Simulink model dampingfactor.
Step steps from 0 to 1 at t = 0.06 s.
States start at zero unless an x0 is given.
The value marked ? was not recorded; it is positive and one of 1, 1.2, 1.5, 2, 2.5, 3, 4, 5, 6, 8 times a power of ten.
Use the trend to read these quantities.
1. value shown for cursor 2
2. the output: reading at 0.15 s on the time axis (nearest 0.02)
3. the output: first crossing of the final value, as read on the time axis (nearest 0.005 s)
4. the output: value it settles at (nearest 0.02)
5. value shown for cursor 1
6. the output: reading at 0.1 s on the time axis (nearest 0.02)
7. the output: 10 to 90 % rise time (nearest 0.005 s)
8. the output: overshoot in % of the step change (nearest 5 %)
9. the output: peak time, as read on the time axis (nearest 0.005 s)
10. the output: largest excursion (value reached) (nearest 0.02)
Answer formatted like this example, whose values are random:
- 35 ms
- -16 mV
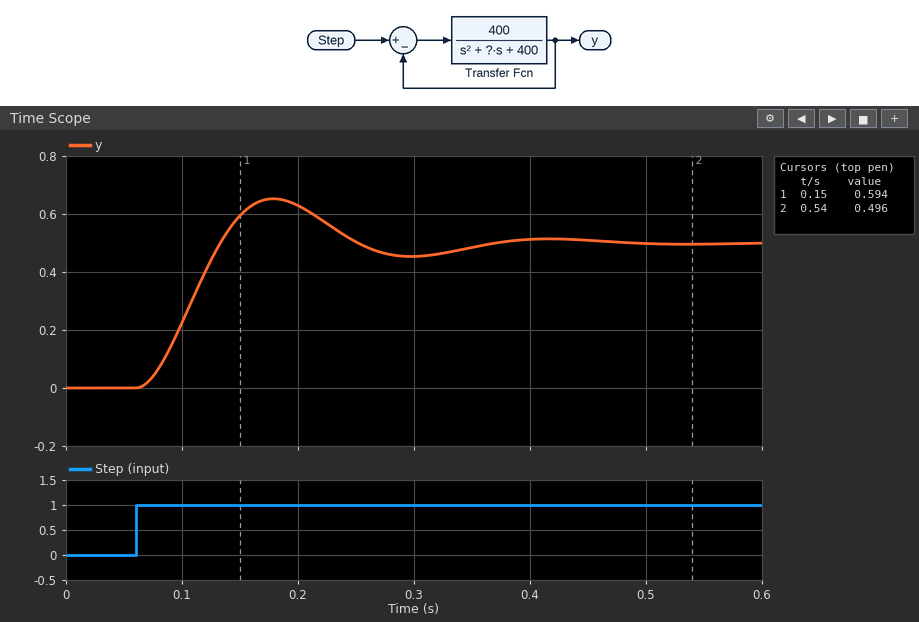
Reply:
- 0.496
- 0.60
- 0.135 s
- 0.50
- 0.594
- 0.22
- 0.050 s
- 30 %
- 0.180 s
- 0.66
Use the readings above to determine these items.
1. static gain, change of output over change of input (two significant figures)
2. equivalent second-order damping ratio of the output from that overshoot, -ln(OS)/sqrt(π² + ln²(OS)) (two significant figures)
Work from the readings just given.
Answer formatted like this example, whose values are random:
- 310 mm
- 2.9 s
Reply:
- 0.50
- 0.36
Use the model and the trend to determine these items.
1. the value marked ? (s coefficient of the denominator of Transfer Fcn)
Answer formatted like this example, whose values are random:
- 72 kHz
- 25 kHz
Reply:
- 20
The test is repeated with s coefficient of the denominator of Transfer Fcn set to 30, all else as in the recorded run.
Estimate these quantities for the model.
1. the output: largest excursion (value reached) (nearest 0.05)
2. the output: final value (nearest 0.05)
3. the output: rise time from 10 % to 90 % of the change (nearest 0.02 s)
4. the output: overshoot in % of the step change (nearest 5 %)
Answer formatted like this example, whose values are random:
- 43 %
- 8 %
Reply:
- 0.55
- 0.50
- 0.06 s
- 15 %
